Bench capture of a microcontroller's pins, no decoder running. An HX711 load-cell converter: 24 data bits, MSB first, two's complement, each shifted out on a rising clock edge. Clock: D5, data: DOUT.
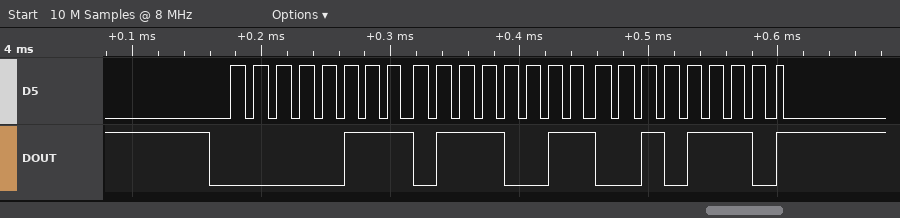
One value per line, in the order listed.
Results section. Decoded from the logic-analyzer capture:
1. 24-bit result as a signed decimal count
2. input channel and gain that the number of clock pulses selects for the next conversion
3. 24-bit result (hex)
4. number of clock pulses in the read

488238
channel A, gain 128
0x07732E
25
